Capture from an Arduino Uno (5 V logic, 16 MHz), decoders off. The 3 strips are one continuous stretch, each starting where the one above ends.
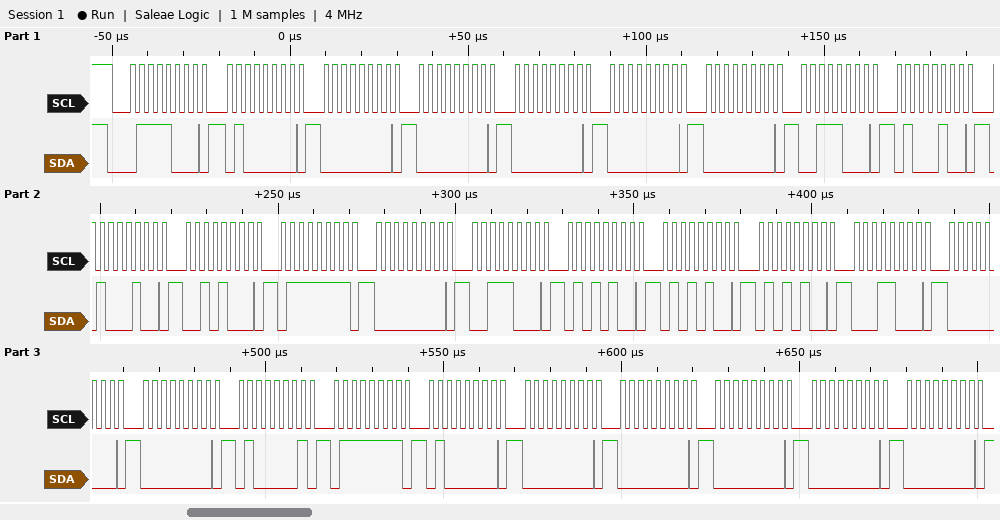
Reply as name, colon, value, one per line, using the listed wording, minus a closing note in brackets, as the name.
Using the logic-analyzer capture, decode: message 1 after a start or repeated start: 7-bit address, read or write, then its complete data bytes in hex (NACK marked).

message 1 after a start or repeated start: 7-bit address, read or write, then its complete data bytes in hex: 0x3C write: 40 00 00 00 00 00 38 44 44 28 7F 00 38 54 54 54 18 00 00 41 7F 40 00 00 00 00 00
